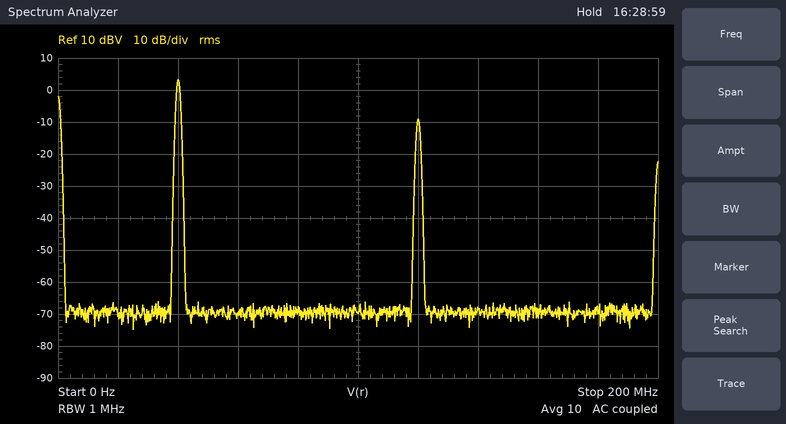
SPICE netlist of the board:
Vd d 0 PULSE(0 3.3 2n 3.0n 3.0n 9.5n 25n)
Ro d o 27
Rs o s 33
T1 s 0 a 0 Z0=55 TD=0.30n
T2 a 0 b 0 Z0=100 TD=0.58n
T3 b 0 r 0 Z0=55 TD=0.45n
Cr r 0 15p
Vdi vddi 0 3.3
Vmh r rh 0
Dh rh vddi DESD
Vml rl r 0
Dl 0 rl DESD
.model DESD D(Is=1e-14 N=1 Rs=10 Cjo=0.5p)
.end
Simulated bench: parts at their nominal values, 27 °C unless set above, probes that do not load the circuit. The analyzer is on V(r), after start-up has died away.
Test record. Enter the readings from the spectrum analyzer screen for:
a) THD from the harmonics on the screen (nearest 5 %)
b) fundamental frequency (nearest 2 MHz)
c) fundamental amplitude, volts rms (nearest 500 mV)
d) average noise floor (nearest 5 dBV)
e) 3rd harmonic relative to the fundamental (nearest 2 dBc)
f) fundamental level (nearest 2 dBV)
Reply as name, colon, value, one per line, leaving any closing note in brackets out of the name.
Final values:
THD from the harmonics on the screen: 25 %
fundamental frequency: 40 MHz
fundamental amplitude, volts rms: 1.5 V
average noise floor: -70 dBV
3rd harmonic relative to the fundamental: -12 dBc
fundamental level: 4 dBV
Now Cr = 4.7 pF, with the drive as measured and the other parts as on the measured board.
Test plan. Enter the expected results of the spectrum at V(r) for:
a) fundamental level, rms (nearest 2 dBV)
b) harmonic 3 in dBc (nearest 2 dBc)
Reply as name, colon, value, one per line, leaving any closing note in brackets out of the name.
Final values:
fundamental level, rms: 4 dBV
harmonic 3 in dBc: -10 dBc
